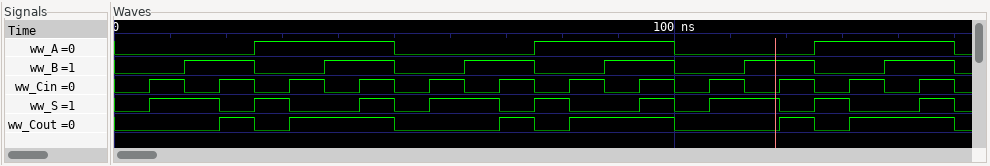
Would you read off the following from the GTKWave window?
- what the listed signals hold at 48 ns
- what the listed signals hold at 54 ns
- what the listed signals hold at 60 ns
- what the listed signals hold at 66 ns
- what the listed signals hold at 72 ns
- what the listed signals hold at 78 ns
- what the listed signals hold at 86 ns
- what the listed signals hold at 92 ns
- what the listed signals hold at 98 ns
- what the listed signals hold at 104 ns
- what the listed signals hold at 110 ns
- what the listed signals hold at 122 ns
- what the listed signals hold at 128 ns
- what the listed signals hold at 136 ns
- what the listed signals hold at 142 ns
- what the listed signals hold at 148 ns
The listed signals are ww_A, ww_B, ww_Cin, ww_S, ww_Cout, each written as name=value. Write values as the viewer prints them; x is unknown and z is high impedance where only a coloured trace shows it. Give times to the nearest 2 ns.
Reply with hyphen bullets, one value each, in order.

- ww_A=1, ww_B=1, ww_Cin=1, ww_S=1, ww_Cout=1
- ww_A=0, ww_B=0, ww_Cin=0, ww_S=0, ww_Cout=0
- ww_A=0, ww_B=0, ww_Cin=1, ww_S=1, ww_Cout=0
- ww_A=0, ww_B=1, ww_Cin=0, ww_S=1, ww_Cout=0
- ww_A=0, ww_B=1, ww_Cin=1, ww_S=0, ww_Cout=1
- ww_A=1, ww_B=0, ww_Cin=0, ww_S=1, ww_Cout=0
- ww_A=1, ww_B=0, ww_Cin=1, ww_S=0, ww_Cout=1
- ww_A=1, ww_B=1, ww_Cin=0, ww_S=0, ww_Cout=1
- ww_A=1, ww_B=1, ww_Cin=1, ww_S=1, ww_Cout=1
- ww_A=0, ww_B=0, ww_Cin=0, ww_S=0, ww_Cout=0
- ww_A=0, ww_B=0, ww_Cin=1, ww_S=1, ww_Cout=0
- ww_A=0, ww_B=1, ww_Cin=1, ww_S=0, ww_Cout=1
- ww_A=1, ww_B=0, ww_Cin=0, ww_S=1, ww_Cout=0
- ww_A=1, ww_B=0, ww_Cin=1, ww_S=0, ww_Cout=1
- ww_A=1, ww_B=1, ww_Cin=0, ww_S=0, ww_Cout=1
- ww_A=1, ww_B=1, ww_Cin=1, ww_S=1, ww_Cout=1
